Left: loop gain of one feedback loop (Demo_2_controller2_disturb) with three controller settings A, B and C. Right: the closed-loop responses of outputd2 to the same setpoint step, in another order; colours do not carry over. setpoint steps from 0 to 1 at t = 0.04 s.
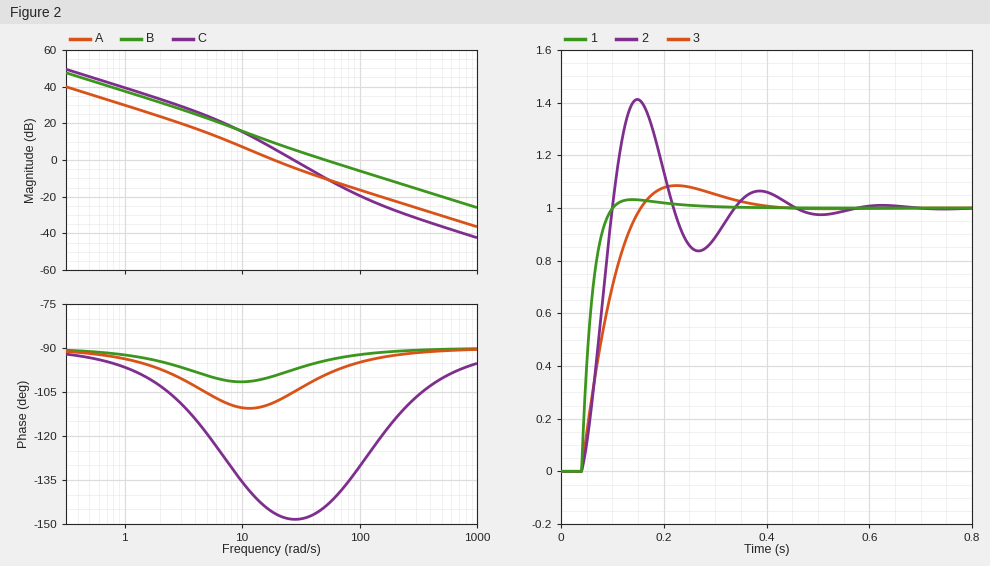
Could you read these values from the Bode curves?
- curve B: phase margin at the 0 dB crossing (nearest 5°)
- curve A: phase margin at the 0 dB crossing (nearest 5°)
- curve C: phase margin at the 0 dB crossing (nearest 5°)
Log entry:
85°
70°
30°
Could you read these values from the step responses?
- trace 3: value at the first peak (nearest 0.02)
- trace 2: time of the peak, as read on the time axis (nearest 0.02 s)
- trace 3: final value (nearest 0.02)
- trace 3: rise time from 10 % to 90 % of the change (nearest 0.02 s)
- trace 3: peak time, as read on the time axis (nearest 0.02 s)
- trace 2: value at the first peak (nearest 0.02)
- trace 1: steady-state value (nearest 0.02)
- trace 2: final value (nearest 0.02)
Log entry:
1.08
0.14 s
1.00
0.08 s
0.22 s
1.42
1.00
1.00
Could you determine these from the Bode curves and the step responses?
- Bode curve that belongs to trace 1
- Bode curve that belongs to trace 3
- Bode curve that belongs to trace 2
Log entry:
B
A
C
